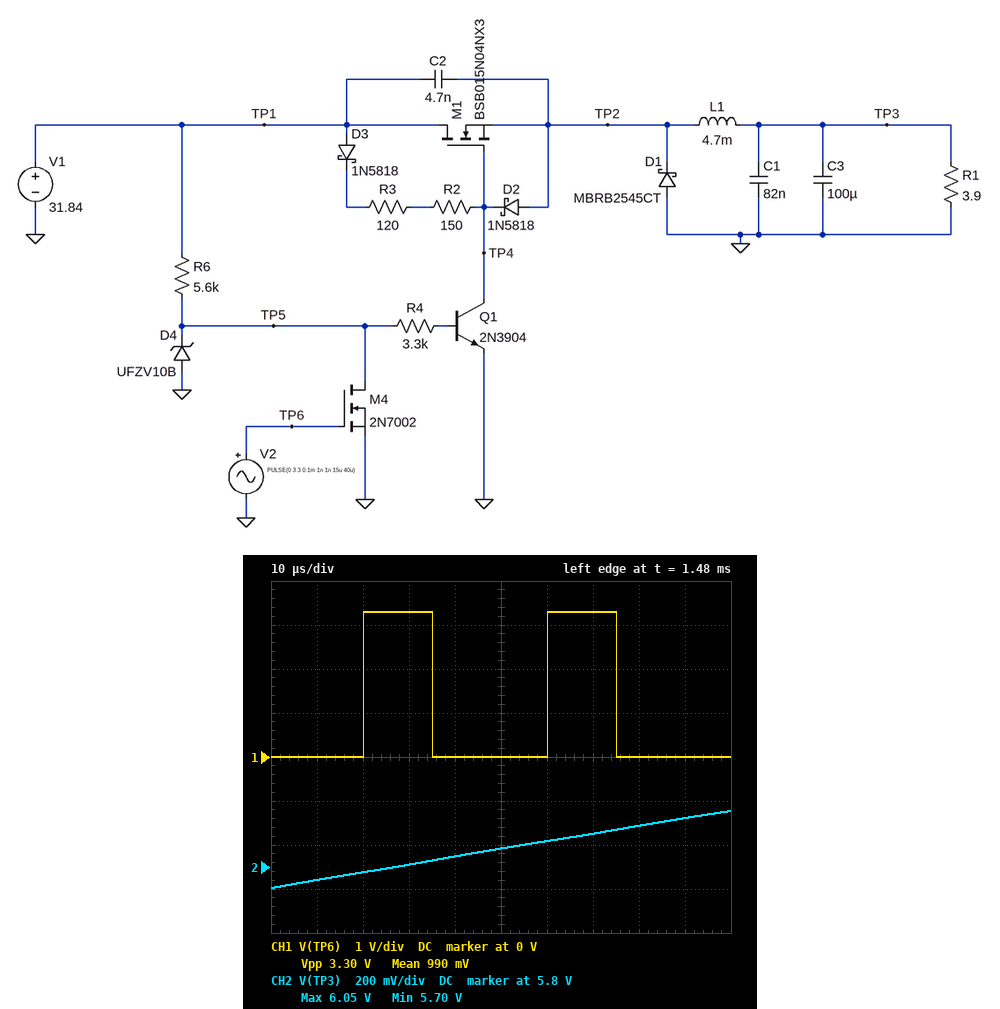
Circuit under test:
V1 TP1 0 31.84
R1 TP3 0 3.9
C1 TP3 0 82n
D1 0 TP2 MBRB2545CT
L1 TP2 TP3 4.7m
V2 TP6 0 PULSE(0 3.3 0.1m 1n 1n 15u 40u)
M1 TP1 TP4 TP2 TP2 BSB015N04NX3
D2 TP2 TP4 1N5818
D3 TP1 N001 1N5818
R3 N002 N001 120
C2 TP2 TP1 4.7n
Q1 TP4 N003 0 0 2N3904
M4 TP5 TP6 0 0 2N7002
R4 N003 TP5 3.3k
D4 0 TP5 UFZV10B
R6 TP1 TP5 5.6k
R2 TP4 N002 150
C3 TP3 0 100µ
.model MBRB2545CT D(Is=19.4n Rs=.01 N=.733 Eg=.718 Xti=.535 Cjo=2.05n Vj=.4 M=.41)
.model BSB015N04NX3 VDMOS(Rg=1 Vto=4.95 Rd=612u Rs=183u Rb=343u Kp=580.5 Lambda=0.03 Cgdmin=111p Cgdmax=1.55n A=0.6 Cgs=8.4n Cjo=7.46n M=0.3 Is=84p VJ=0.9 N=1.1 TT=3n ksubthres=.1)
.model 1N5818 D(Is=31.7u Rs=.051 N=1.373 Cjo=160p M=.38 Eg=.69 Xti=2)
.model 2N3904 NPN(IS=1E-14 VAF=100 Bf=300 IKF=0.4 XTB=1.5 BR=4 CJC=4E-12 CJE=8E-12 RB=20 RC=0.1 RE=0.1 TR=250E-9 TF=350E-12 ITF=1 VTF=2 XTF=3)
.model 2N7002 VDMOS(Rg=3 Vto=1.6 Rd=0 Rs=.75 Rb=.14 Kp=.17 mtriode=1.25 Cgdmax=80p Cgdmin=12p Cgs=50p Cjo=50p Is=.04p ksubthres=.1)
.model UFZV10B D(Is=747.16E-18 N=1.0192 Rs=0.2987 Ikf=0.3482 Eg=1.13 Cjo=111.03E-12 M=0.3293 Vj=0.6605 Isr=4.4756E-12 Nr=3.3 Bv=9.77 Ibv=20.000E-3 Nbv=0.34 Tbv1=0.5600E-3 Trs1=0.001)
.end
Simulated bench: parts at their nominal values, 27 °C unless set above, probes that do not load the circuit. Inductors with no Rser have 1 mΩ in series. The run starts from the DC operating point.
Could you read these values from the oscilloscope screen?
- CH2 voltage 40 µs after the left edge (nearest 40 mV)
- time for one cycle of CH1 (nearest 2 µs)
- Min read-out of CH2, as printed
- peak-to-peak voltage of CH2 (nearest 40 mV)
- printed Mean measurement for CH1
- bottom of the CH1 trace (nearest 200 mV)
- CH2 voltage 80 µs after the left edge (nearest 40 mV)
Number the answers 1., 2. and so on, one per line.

1. 5.84 V
2. 40 µs
3. 5.70 V
4. 360 mV
5. 990 mV
6. 0 V
7. 6.00 V
